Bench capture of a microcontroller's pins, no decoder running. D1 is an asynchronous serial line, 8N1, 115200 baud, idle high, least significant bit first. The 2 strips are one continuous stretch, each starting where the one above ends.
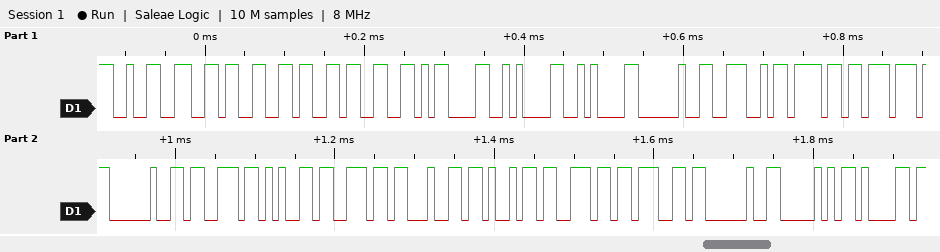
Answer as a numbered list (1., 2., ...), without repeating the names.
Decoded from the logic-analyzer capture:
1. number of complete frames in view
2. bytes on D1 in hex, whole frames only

1. 22
2. 0x32 0x36 0x36 0x33 0x0D 0x0A 0x0A 0x20 0x4E 0x6F 0x77 0x20 0x73 0x65 0x6E 0x64 0x69 0x6E 0x67 0x20 0x50 0x61
